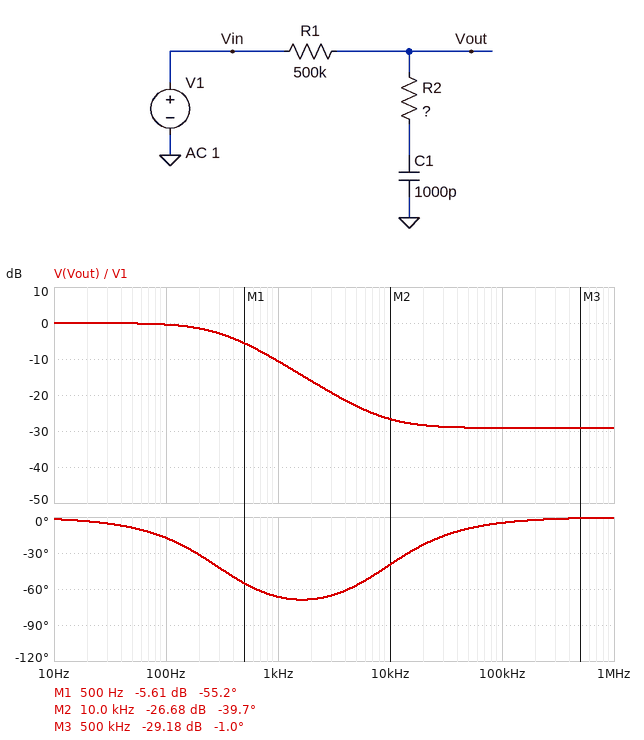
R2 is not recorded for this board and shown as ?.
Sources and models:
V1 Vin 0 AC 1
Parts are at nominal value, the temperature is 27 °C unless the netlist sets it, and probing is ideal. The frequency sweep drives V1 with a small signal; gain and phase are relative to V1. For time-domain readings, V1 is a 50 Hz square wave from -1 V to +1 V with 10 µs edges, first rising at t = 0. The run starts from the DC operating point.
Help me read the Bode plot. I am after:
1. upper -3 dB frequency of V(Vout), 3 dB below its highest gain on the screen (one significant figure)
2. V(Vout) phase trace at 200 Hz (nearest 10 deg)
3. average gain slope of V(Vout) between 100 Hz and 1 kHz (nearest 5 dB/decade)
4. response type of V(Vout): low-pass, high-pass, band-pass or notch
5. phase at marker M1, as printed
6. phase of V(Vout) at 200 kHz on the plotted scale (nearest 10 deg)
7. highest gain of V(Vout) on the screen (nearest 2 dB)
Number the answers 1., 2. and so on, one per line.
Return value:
1. 300 Hz
2. -30 deg
3. -10 dB/decade
4. low-pass
5. -55.2 deg
6. 0 deg
7. 0 dB
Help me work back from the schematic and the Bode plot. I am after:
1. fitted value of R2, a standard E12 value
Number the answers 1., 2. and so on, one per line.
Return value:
1. 18 kΩ
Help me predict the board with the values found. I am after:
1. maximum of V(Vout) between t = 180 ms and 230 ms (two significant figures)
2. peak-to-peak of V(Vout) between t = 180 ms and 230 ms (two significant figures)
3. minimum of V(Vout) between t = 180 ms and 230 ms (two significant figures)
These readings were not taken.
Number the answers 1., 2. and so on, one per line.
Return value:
1. 1.0 V
2. 2.0 V
3. -1.0 V
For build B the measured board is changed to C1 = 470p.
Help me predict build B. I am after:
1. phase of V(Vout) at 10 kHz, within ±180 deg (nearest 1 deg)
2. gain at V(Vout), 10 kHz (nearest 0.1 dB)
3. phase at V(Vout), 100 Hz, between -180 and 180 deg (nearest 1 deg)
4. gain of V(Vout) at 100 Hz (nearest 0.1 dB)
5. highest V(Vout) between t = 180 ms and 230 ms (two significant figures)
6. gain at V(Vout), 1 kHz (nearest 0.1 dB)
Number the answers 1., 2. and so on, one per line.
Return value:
1. -58 deg
2. -22.6 dB
3. -8 deg
4. -0.1 dB
5. 1.0 V
6. -5.2 dB
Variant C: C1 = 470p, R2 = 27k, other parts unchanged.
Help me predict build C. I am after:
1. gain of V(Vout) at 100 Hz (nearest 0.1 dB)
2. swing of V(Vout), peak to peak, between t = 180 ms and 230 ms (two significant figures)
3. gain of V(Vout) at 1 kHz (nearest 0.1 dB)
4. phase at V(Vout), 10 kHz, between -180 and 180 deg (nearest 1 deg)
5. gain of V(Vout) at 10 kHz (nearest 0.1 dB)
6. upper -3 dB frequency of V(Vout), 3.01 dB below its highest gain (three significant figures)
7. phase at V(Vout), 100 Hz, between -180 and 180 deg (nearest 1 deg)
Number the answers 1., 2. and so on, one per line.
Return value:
1. -0.1 dB
2. 2.0 V
3. -5.3 dB
4. -48 deg
5. -21.7 dB
6. 644 Hz
7. -8 deg
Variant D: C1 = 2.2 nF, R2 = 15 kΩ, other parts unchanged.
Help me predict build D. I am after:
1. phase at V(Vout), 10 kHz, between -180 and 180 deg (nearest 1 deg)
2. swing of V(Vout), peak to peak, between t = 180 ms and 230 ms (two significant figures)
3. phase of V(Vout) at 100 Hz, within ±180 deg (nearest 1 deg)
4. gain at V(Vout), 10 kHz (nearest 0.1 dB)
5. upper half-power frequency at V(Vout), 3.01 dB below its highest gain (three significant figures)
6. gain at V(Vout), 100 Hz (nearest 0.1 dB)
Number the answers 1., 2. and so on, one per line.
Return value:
1. -25 deg
2. 2.0 V
3. -34 deg
4. -29.8 dB
5. 141 Hz
6. -1.8 dB
